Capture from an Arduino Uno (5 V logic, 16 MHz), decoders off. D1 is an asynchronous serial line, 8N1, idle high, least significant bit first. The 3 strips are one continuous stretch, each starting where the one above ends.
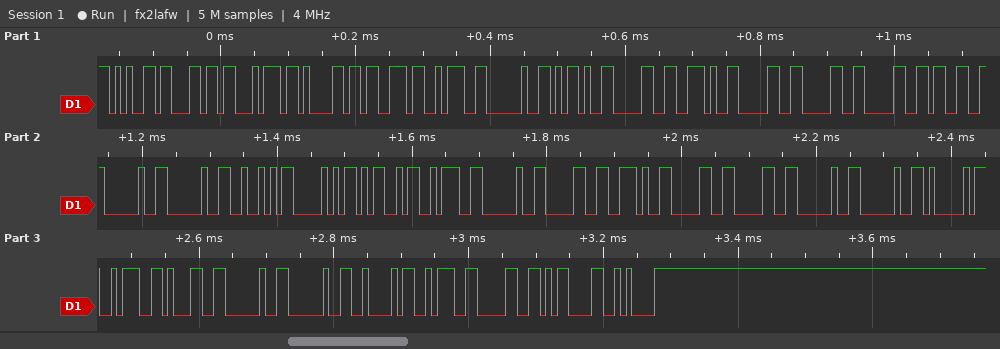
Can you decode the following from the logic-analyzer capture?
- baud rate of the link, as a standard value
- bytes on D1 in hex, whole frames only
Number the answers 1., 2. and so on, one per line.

1. 115200 baud
2. 65 6C 74 61 73 3A 20 2D 30 2E 30 30 30 33 20 20 52 50 4D 3A 20 30 2E 30 30 20 20 41 3A 31 20 20 42 3A 30 0D 0A
